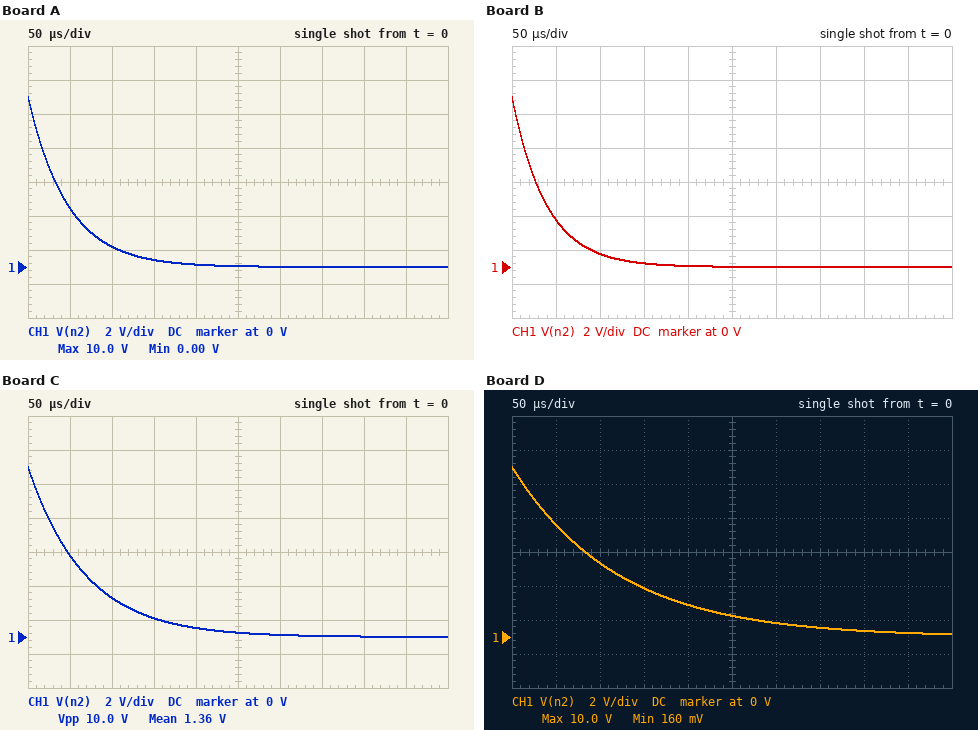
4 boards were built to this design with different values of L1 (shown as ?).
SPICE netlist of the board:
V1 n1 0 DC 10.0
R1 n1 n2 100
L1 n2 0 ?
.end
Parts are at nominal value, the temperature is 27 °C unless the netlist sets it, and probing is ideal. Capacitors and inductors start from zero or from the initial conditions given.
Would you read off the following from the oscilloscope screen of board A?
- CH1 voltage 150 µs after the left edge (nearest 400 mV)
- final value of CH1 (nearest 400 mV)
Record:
400 mV
0 V
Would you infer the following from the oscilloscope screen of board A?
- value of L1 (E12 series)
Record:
4.7 mH
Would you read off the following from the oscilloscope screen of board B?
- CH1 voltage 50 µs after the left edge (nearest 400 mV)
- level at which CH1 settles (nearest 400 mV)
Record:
2.8 V
0 V
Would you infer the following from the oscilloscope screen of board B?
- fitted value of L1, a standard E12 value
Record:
3.9 mH
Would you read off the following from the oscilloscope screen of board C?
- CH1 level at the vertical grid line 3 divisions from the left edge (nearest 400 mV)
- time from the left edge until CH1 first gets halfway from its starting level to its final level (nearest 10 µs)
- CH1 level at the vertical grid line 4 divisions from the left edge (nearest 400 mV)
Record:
1.2 V
50 µs
400 mV
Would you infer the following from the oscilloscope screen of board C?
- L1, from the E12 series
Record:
6.8 mH
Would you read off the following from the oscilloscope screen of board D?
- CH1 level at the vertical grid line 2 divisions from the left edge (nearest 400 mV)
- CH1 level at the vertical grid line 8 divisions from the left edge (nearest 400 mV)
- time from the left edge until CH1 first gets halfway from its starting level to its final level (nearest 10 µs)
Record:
4.4 V
400 mV
80 µs
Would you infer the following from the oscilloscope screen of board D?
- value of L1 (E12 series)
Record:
12 mH
